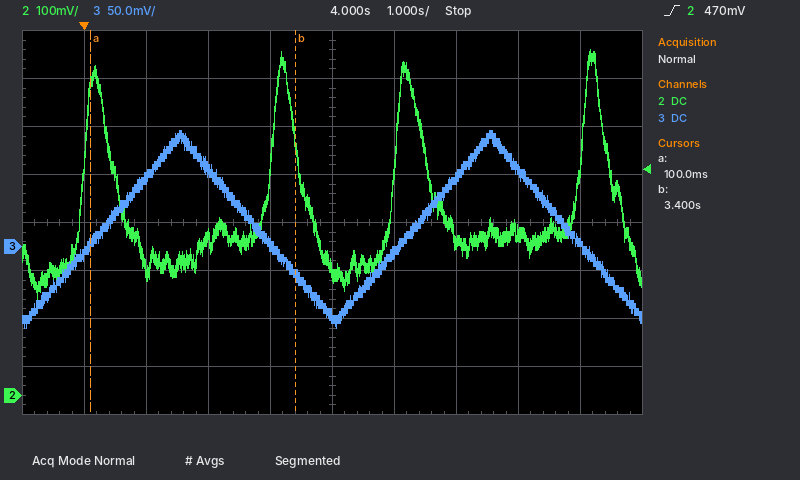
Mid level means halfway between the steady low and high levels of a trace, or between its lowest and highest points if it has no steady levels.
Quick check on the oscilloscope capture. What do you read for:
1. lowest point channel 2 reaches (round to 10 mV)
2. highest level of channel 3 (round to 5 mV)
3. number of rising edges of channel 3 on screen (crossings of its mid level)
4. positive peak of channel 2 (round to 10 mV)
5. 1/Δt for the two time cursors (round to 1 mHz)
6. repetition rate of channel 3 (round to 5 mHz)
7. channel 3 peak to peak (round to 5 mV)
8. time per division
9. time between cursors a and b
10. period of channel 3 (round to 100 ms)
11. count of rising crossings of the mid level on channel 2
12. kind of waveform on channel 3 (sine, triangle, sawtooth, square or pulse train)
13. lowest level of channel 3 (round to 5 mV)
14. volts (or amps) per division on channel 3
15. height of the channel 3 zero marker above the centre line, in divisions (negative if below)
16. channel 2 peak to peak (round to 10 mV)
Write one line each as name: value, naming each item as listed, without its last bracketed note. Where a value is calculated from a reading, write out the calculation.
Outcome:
lowest point channel 2 reaches: 200 mV
highest level of channel 3: 120 mV
number of rising edges of channel 3 on screen: 2
positive peak of channel 2: 720 mV
1/Δt for the two time cursors: 1 / 3.3 s ≈ 303 mHz
repetition rate of channel 3: 1 / 5.0 s ≈ 200 mHz
channel 3 peak to peak: 120 mV − (-85 mV) = 205 mV
time per division: 1 s
time between cursors a and b: 3.4 s − (100 ms) = 3.3 s
period of channel 3: 5.0 s
count of rising crossings of the mid level on channel 2: 4
kind of waveform on channel 3: triangle
lowest level of channel 3: -85 mV
volts (or amps) per division on channel 3: 50 mV
height of the channel 3 zero marker above the centre line, in divisions: -0.5 div
channel 2 peak to peak: 720 mV − (200 mV) = 520 mV
